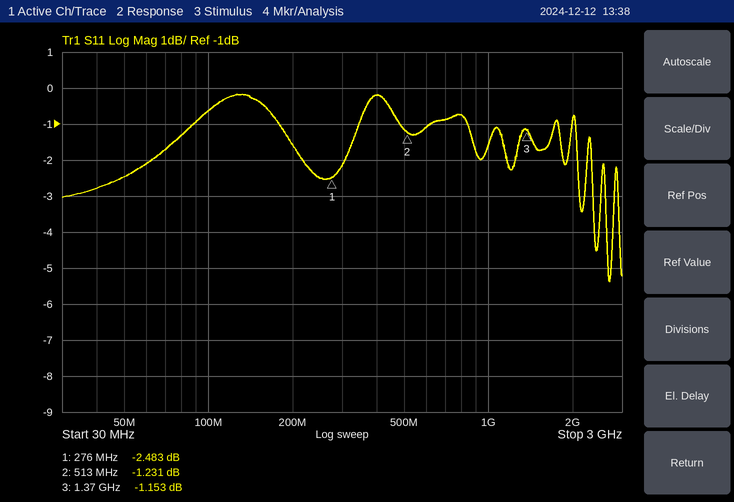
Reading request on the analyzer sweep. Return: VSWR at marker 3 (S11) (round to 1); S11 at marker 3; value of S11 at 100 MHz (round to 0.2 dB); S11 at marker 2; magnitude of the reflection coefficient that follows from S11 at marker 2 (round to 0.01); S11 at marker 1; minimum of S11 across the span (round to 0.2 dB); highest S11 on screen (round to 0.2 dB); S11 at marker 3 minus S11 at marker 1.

15
-1.153 dB
-0.6 dB
-1.231 dB
0.87
-2.483 dB
-5.4 dB
-0.2 dB
1.330 dB
